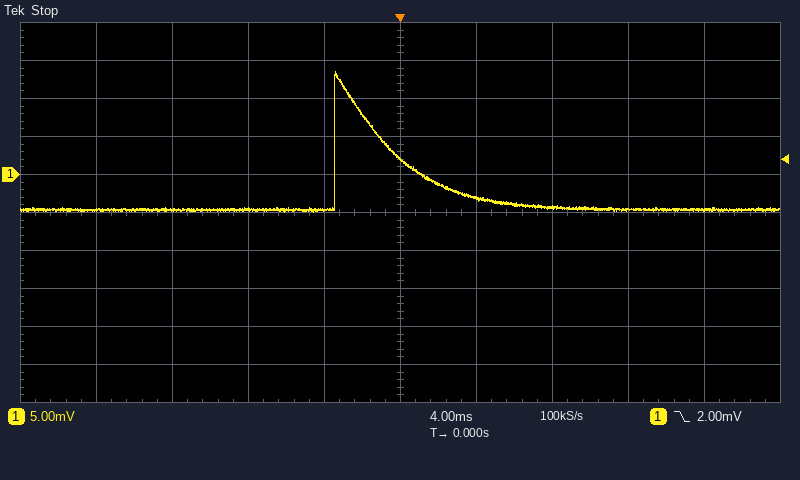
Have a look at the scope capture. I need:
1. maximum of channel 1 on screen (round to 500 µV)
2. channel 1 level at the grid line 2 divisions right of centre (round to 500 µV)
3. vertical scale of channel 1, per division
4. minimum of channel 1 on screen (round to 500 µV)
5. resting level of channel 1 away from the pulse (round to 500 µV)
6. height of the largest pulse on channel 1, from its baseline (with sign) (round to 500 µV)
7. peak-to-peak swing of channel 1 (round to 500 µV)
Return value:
13.5 mV
-4.5 mV
5 mV
-5.0 mV
-4.5 mV
+18.0 mV
18.5 mV
